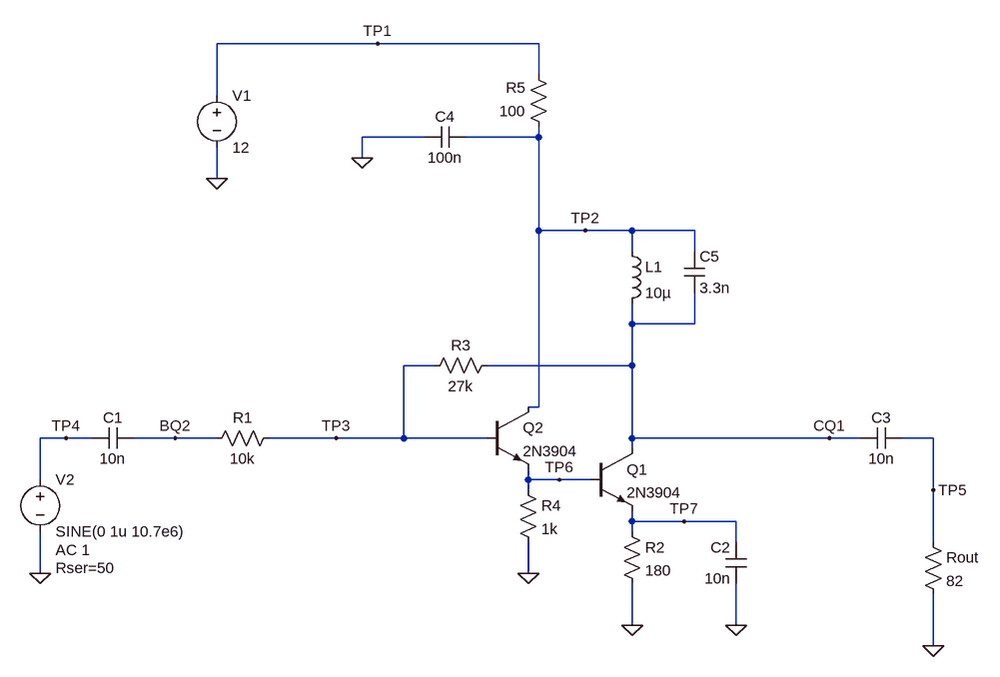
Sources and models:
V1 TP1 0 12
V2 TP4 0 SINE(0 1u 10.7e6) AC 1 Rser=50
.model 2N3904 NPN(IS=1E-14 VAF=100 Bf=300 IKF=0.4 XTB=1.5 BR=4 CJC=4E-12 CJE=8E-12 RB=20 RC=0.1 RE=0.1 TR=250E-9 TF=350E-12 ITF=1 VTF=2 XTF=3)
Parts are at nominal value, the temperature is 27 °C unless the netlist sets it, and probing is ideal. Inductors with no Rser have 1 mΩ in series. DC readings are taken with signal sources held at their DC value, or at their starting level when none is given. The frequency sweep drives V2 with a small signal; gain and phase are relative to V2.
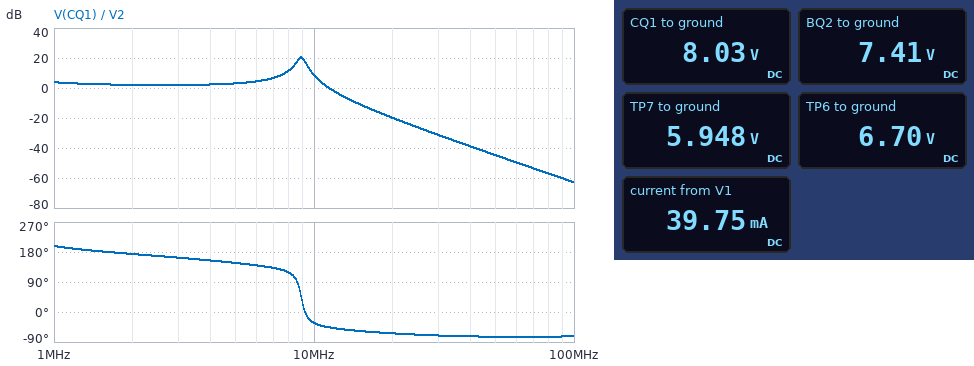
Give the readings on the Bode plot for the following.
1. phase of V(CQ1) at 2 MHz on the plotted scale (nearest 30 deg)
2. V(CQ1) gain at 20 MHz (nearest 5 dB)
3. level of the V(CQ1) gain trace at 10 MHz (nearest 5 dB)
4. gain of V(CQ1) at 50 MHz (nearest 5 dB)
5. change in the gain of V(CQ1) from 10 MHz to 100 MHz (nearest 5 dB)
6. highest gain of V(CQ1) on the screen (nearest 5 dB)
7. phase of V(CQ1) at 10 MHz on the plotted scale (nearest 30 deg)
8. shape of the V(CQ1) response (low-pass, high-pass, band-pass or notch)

180 deg
-20 dB
10 dB
-45 dB
-70 dB
20 dB
-30 deg
low-pass
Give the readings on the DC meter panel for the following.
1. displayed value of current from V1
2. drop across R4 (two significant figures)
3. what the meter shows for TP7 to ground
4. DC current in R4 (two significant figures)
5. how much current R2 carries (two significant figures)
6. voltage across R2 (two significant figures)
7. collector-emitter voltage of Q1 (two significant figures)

39.75 mA
6.7 V
5.948 V
6.7 mA
33 mA
5.9 V
2.1 V
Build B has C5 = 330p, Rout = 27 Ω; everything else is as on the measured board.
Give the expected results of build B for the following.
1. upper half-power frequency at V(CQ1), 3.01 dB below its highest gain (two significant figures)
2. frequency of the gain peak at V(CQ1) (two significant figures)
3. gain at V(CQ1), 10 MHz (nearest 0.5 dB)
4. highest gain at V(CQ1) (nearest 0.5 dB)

13 MHz
12 MHz
13.5 dB
23.0 dB
